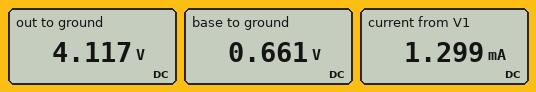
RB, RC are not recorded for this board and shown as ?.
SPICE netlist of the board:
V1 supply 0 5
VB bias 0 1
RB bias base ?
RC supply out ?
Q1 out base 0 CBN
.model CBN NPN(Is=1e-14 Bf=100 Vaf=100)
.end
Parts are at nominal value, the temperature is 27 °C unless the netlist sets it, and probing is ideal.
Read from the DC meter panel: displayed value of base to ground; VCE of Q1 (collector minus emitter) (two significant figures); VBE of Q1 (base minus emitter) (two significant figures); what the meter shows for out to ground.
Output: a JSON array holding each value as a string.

["0.661 V", "4.1 V", "660 mV", "4.117 V"]
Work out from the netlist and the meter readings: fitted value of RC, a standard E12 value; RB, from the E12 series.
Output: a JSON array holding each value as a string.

["680 Ω", "27 kΩ"]
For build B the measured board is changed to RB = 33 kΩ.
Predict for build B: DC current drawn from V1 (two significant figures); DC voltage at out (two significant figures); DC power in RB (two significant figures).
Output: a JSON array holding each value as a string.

["1.1 mA", "4.3 V", "3.6 µW"]
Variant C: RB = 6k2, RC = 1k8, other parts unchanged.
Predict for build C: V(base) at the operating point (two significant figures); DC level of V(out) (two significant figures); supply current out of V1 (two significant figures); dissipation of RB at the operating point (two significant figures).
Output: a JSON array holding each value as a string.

["680 mV", "120 mV", "2.7 mA", "16 µW"]
